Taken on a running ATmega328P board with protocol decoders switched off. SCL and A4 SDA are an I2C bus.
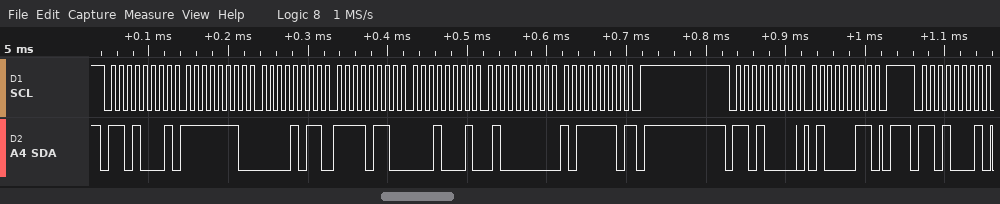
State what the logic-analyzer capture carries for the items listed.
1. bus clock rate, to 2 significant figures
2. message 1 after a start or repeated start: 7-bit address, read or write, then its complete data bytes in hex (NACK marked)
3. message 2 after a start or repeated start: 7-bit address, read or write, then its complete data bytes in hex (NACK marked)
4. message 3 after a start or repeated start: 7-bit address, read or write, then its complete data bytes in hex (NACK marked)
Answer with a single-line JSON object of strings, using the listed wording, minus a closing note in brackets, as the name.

{"bus clock rate, to 2 significant figures": "100 kHz", "message 1 after a start or repeated start: 7-bit address, read or write, then its complete data bytes in hex": "0x68 read: FE 0B F6 11 40 BE NACK", "message 2 after a start or repeated start: 7-bit address, read or write, then its complete data bytes in hex": "0x68 write: 43", "message 3 after a start or repeated start: 7-bit address, read or write, then its complete data bytes in hex": "0x68 read"}
